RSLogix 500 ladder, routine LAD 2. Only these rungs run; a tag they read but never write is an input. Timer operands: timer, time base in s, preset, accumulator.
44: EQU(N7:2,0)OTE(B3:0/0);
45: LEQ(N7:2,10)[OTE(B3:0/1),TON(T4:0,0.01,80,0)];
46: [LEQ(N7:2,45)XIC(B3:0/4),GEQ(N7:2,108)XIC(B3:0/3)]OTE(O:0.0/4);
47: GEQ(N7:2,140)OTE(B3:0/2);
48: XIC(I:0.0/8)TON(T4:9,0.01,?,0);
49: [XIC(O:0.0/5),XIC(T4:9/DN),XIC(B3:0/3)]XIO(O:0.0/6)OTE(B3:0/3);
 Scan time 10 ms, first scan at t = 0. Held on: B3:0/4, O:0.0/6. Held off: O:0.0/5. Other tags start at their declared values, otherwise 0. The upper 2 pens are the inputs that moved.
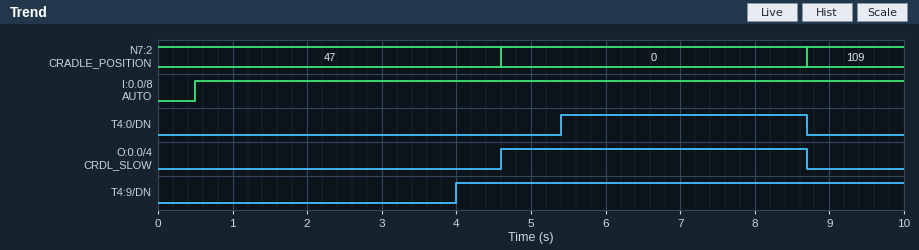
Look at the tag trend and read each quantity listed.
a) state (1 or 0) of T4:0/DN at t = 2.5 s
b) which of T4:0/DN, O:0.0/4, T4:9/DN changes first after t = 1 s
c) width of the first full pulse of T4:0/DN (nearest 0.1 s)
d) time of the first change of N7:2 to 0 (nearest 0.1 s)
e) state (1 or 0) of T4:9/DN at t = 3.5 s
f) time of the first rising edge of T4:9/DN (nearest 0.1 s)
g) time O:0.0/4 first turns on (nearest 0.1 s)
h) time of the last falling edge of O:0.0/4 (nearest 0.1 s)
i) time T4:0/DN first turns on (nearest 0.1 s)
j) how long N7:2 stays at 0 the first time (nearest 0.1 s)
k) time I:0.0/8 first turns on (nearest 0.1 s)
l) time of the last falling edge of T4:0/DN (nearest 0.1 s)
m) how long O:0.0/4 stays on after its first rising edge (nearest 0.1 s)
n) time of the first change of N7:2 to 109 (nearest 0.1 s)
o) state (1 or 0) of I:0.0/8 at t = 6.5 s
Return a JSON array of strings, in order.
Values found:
["0", "T4:9/DN", "3.3 s", "4.6 s", "0", "4.0 s", "4.6 s", "8.7 s", "5.4 s", "4.1 s", "0.5 s", "8.7 s", "4.1 s", "8.7 s", "1"]
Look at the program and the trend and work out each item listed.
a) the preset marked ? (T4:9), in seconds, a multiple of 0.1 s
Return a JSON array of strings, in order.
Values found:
["3.5 s"]
